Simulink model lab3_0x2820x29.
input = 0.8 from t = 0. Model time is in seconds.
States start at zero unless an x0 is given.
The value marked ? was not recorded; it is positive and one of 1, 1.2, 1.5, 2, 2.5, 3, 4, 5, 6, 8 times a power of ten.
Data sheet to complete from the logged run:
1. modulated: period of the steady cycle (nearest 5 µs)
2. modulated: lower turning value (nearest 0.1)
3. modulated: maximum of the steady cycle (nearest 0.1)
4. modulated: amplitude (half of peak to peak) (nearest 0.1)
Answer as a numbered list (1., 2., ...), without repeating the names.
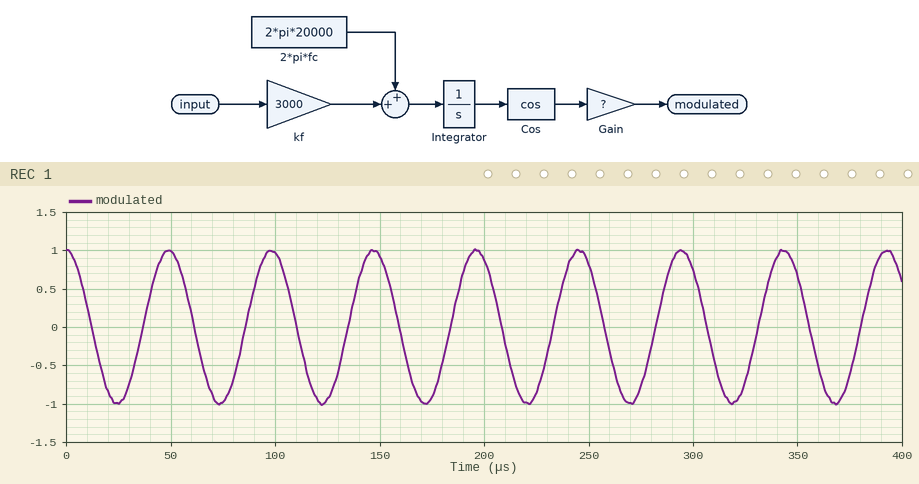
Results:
1. 50 µs
2. -1.0
3. 1.0
4. 1.0
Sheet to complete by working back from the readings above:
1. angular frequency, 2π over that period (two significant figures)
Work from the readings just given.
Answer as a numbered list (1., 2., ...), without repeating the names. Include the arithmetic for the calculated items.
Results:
1. 2π / 50 = 0.13 rad/µs
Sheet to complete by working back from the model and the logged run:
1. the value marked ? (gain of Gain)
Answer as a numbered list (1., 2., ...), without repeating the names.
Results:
1. 1
